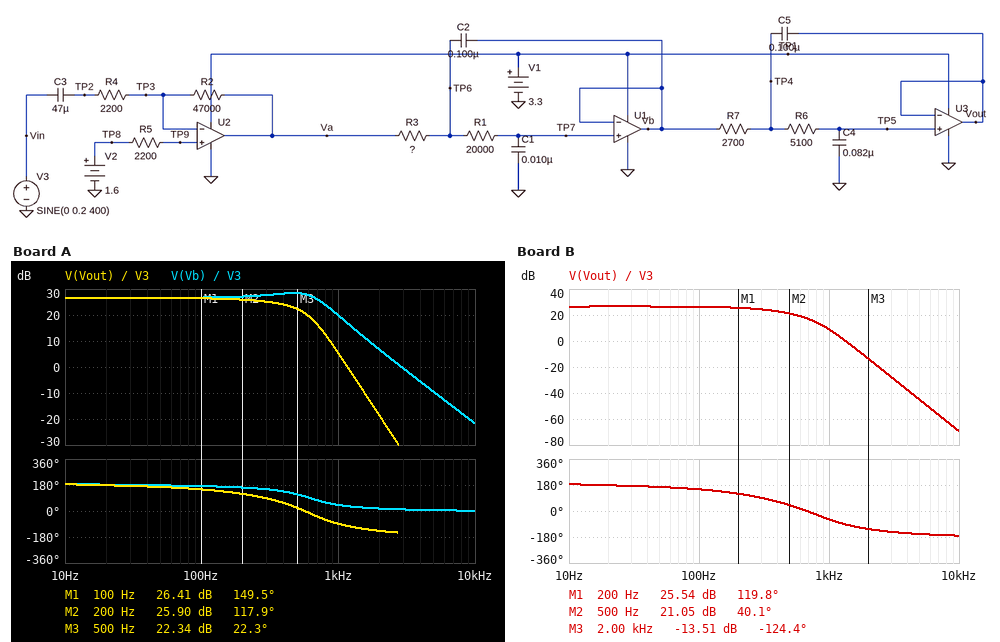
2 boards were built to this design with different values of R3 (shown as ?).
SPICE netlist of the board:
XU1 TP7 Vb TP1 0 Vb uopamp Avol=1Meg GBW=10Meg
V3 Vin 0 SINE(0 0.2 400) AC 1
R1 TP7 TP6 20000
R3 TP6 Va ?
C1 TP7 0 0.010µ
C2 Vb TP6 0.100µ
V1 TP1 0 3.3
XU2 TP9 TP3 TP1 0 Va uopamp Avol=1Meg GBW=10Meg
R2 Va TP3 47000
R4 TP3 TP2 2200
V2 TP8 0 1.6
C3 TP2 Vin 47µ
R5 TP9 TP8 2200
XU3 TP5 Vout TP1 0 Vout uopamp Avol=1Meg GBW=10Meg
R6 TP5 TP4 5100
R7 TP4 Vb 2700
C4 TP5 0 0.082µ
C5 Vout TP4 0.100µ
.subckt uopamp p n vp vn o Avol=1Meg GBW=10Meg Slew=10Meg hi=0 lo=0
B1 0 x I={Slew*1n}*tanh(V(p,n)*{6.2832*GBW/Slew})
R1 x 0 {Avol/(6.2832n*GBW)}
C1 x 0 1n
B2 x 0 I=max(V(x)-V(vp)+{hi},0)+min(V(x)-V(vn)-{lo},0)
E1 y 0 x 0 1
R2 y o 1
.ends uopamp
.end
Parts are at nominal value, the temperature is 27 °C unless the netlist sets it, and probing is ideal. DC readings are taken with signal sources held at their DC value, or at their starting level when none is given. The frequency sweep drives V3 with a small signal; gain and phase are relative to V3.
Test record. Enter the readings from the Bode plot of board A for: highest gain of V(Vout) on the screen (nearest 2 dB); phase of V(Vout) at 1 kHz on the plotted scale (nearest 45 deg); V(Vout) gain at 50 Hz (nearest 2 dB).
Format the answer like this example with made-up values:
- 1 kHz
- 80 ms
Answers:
- 26 dB
- -90 deg
- 26 dB
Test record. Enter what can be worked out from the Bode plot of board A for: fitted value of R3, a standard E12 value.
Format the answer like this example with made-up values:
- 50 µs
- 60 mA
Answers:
- 3.3 kΩ
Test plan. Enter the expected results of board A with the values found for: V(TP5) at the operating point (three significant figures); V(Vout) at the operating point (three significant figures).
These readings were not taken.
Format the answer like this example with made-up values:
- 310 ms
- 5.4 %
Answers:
- 1.60 V
- 1.60 V
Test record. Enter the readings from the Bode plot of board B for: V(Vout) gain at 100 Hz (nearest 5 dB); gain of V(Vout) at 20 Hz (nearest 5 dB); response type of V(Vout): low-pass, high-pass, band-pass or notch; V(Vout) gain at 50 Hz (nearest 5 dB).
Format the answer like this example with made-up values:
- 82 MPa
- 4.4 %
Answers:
- 25 dB
- 25 dB
- low-pass
- 25 dB
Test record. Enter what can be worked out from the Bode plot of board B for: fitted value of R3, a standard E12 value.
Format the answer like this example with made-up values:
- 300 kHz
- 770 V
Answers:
- 1.8 kΩ
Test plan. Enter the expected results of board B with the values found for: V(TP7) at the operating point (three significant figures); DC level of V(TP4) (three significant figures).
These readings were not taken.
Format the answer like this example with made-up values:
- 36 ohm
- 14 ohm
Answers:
- 1.60 V
- 1.60 V
